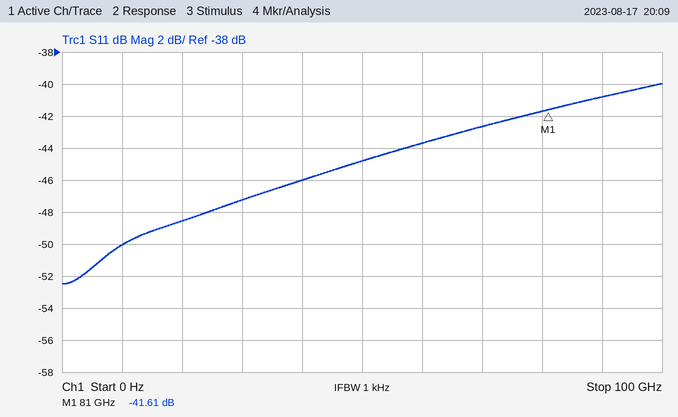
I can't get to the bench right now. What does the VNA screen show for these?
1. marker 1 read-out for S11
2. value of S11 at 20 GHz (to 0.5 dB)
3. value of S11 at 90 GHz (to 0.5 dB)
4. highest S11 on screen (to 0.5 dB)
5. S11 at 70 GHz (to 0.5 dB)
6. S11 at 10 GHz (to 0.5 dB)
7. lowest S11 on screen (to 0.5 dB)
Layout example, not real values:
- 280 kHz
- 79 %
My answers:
- -41.61 dB
- -48.5 dB
- -41.0 dB
- -40.0 dB
- -42.5 dB
- -50.0 dB
- -52.5 dB
